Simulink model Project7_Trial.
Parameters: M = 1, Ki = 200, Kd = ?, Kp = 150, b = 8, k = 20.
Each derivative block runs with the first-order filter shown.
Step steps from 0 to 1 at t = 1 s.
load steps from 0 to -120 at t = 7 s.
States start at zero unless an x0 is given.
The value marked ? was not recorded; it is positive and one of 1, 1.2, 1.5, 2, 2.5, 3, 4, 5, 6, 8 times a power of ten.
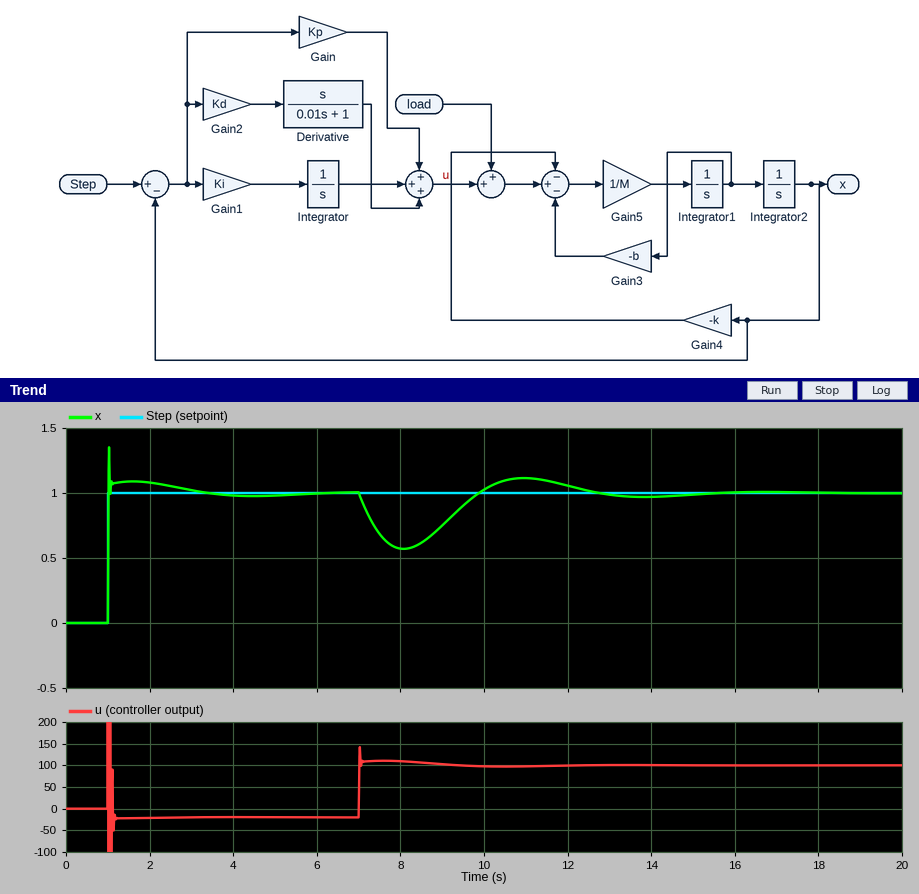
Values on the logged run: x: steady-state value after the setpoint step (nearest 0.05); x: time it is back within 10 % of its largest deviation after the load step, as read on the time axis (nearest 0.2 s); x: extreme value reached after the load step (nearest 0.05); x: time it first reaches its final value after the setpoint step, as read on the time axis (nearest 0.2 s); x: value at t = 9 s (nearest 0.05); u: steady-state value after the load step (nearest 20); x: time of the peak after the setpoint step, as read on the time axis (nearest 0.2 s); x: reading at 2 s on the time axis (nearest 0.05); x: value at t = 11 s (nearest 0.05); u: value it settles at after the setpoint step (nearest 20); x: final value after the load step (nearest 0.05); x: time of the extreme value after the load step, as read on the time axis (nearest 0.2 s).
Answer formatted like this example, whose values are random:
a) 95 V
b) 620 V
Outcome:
a) 1.00
b) 12.2 s
c) 0.55
d) 1.0 s
e) 0.75
f) 100
g) 1.0 s
h) 1.10
i) 1.10
j) -20
k) 1.00
l) 8.0 s
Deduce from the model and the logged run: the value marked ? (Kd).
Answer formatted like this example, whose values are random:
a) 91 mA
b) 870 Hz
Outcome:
a) 150
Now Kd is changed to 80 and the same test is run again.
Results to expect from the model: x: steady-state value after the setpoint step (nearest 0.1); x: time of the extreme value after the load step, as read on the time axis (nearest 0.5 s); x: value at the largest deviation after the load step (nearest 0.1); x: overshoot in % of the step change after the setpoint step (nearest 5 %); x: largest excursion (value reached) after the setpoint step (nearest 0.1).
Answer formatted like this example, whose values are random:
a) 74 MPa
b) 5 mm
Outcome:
a) 1.0
b) 7.5 s
c) 0.5
d) 30 %
e) 1.3
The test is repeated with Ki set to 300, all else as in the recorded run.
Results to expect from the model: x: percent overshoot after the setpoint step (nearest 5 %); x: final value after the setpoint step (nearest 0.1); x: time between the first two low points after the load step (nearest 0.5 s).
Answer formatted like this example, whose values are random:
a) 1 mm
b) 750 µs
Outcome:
a) 35 %
b) 1.0
c) 4.5 s
